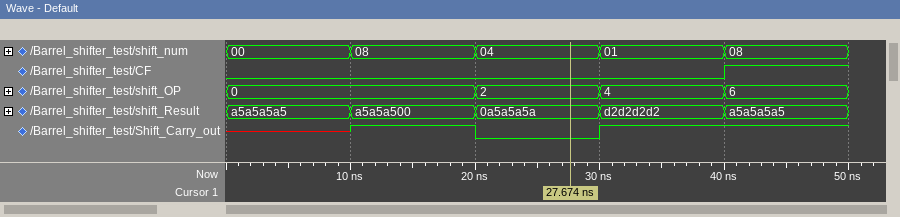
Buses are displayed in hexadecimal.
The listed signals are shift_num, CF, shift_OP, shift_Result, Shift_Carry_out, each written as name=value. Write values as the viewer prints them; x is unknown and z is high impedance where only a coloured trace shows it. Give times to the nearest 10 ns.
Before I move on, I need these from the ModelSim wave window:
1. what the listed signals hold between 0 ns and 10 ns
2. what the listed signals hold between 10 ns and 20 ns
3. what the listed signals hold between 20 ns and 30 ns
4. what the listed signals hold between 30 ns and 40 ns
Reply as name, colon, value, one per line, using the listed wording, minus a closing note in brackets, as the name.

what the listed signals hold between 0 ns and 10 ns: shift_num=00, CF=0, shift_OP=0, shift_Result=a5a5a5a5, Shift_Carry_out=x
what the listed signals hold between 10 ns and 20 ns: shift_num=08, CF=0, shift_OP=0, shift_Result=a5a5a500, Shift_Carry_out=1
what the listed signals hold between 20 ns and 30 ns: shift_num=04, CF=0, shift_OP=2, shift_Result=0a5a5a5a, Shift_Carry_out=0
what the listed signals hold between 30 ns and 40 ns: shift_num=01, CF=0, shift_OP=4, shift_Result=d2d2d2d2, Shift_Carry_out=1
